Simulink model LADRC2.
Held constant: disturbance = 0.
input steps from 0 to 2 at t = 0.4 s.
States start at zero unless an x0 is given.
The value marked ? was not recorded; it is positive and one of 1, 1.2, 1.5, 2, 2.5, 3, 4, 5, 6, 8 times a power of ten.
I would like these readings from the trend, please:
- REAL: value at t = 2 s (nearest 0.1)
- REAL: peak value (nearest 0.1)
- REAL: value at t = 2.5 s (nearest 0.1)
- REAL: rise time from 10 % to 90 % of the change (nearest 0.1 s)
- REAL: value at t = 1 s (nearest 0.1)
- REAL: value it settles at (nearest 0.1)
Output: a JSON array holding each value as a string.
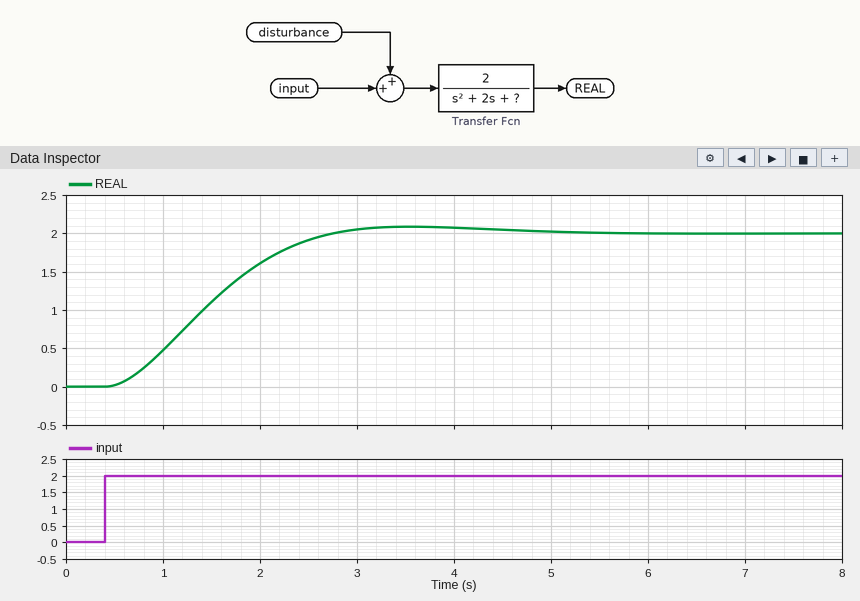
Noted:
["1.6", "2.1", "1.9", "1.5 s", "0.5", "2.0"]
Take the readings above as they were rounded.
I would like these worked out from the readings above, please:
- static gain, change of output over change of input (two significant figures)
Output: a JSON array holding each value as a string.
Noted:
["1.0"]
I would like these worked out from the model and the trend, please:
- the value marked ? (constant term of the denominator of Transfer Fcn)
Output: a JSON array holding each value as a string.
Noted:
["2"]
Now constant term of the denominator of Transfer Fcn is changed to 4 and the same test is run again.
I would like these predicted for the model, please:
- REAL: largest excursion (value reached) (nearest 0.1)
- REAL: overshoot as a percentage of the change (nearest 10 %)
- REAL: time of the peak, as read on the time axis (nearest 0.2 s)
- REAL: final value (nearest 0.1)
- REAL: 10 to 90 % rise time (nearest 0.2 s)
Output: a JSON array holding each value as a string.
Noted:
["1.2", "20 %", "2.2 s", "1.0", "0.8 s"]
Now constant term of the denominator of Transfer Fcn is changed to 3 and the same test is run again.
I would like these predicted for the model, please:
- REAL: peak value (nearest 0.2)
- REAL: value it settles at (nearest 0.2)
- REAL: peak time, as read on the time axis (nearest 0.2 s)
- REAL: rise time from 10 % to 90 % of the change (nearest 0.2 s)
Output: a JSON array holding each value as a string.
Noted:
["1.4", "1.4", "2.6 s", "1.0 s"]
